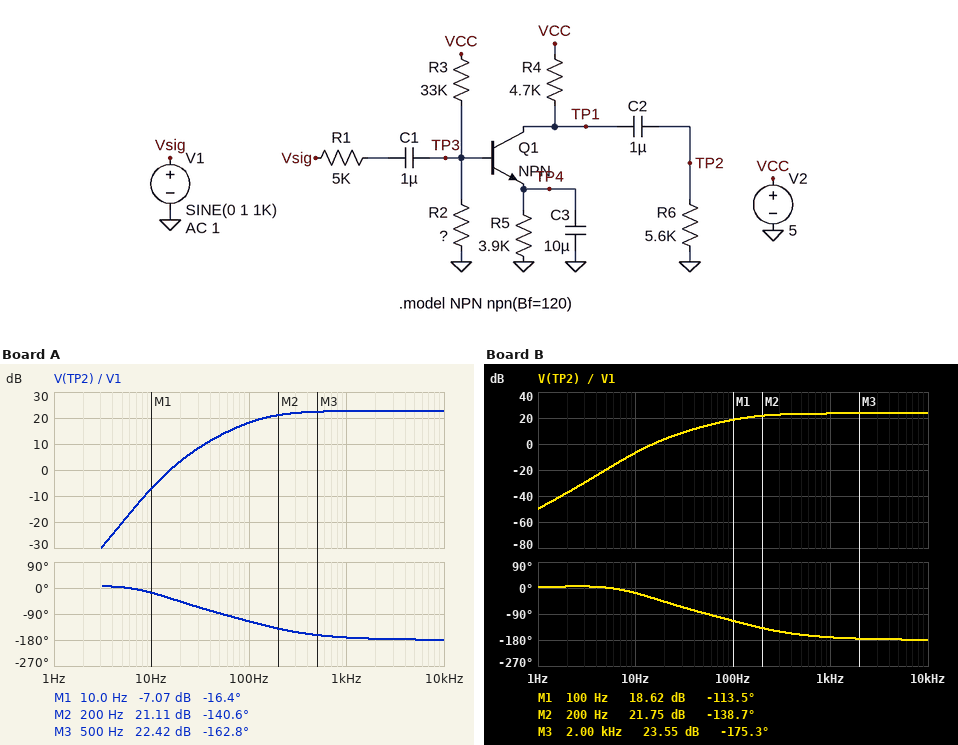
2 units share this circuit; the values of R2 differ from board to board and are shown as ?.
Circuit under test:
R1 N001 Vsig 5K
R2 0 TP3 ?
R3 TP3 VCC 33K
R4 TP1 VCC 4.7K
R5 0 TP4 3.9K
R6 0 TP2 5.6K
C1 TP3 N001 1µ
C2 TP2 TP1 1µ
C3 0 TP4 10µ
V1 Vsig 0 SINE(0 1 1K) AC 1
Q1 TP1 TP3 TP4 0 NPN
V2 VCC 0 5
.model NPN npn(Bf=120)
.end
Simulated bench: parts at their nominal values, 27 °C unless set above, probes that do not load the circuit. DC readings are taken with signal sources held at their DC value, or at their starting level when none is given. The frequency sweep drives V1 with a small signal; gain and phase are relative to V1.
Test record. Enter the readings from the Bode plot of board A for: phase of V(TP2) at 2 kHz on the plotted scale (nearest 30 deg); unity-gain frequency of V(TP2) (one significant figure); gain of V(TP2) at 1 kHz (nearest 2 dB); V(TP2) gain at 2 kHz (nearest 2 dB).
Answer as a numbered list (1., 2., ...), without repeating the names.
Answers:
1. -180 deg
2. 20 Hz
3. 22 dB
4. 22 dB
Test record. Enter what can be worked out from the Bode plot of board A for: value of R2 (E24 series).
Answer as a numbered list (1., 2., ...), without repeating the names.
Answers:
1. 18 kΩ
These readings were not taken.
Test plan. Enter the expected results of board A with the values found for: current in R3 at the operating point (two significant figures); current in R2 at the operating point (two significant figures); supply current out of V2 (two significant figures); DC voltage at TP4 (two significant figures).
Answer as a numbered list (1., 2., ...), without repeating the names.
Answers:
1. 99 µA
2. 97 µA
3. 350 µA
4. 1.0 V
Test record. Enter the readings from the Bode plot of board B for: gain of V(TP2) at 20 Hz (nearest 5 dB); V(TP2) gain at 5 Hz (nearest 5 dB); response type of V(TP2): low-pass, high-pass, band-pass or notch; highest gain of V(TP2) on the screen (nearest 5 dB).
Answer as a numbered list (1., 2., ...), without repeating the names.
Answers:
1. 5 dB
2. -20 dB
3. high-pass
4. 25 dB
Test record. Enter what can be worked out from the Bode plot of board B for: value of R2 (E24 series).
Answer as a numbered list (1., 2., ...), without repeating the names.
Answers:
1. 20 kΩ
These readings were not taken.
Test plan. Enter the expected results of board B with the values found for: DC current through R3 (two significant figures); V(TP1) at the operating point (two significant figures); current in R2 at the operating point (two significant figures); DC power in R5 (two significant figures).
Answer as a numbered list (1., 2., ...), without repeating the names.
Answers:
1. 95 µA
2. 3.7 V
3. 93 µA
4. 320 µW
